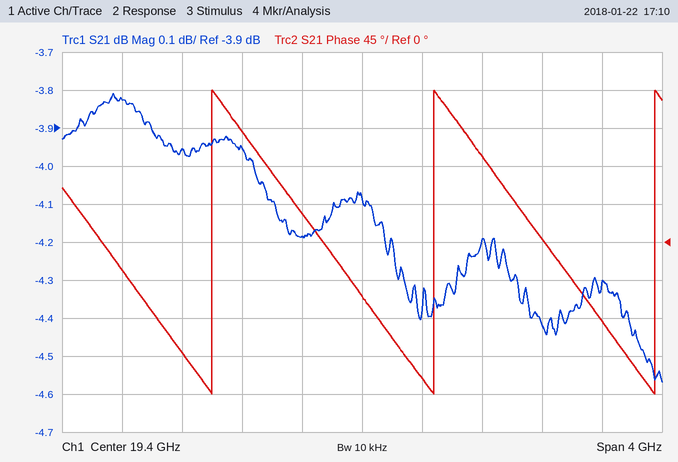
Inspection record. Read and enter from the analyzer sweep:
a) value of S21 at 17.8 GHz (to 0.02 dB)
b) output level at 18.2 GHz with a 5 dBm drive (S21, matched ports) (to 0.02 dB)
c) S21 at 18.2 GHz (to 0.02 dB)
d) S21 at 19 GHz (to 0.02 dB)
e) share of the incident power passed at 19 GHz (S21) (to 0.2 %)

-3.82 dB
1.04 dBm
-3.96 dB
-4.18 dB
38.2 %
